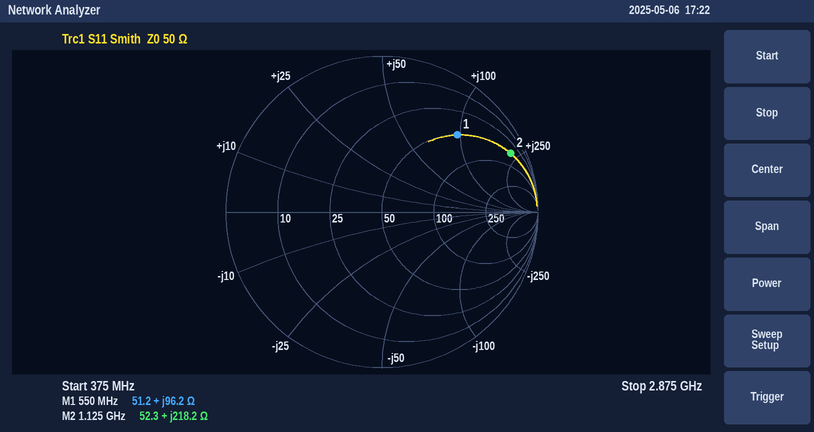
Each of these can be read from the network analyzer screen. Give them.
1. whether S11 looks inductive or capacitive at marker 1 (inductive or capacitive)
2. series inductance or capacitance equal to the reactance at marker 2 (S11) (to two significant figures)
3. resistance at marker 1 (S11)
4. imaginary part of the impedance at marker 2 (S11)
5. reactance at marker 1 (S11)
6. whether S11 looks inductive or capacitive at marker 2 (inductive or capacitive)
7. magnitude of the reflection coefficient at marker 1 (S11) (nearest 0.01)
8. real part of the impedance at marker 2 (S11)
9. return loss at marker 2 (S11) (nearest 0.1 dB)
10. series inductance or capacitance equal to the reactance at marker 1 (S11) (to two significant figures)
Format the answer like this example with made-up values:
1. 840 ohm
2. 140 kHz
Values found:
1. inductive
2. 31 nH
3. 51.2 Ω
4. +218.2 Ω
5. +96.2 Ω
6. inductive
7. 0.69
8. 52.3 Ω
9. 0.9 dB
10. 28 nH
